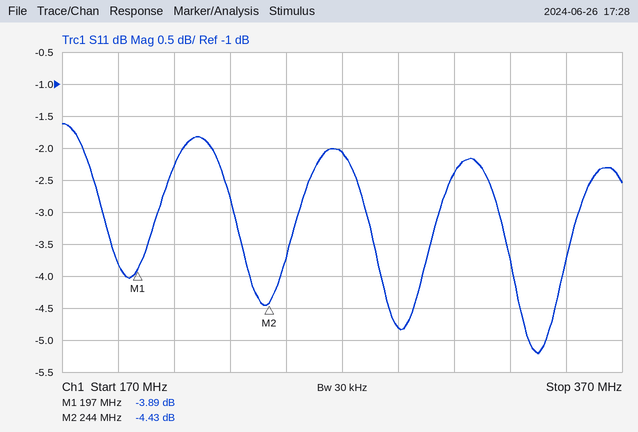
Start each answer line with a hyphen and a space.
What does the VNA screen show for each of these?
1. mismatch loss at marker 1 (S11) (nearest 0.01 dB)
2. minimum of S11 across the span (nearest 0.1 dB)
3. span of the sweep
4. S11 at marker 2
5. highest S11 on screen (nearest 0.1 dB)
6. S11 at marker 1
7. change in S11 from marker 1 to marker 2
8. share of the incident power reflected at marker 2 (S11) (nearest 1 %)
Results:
- 2.28 dB
- -5.2 dB
- 200 MHz
- -4.43 dB
- -1.6 dB
- -3.89 dB
- -0.54 dB
- 36 %
